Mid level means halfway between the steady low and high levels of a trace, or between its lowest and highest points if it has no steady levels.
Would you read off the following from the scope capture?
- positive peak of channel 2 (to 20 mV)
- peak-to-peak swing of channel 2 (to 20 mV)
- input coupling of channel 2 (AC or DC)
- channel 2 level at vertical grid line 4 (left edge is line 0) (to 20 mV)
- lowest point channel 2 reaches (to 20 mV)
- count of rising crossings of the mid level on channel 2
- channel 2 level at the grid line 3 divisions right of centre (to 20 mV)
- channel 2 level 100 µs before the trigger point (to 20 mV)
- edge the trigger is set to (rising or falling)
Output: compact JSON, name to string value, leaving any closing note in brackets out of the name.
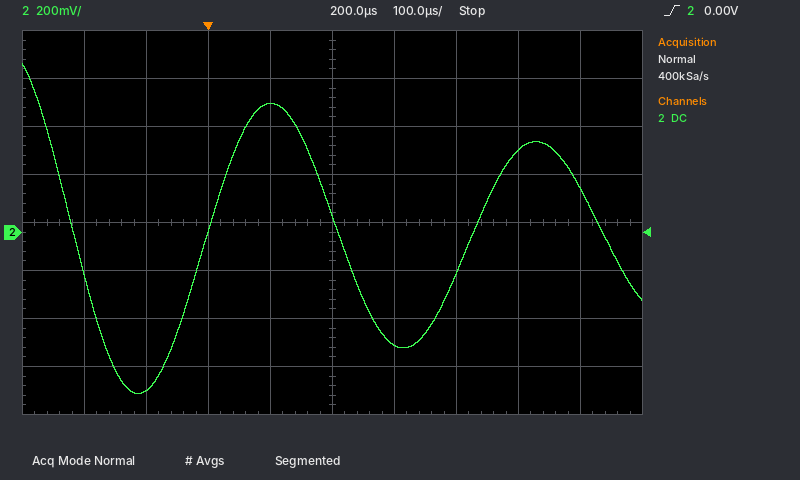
{"positive peak of channel 2": "700 mV", "peak-to-peak swing of channel 2": "1.38 V", "input coupling of channel 2": "DC", "channel 2 level at vertical grid line 4 (left edge is line 0)": "540 mV", "lowest point channel 2 reaches": "-680 mV", "count of rising crossings of the mid level on channel 2": "2", "channel 2 level at the grid line 3 divisions right of centre": "340 mV", "channel 2 level 100 µs before the trigger point": "-660 mV", "edge the trigger is set to": "rising"}
